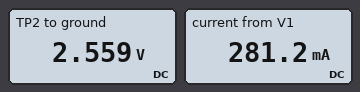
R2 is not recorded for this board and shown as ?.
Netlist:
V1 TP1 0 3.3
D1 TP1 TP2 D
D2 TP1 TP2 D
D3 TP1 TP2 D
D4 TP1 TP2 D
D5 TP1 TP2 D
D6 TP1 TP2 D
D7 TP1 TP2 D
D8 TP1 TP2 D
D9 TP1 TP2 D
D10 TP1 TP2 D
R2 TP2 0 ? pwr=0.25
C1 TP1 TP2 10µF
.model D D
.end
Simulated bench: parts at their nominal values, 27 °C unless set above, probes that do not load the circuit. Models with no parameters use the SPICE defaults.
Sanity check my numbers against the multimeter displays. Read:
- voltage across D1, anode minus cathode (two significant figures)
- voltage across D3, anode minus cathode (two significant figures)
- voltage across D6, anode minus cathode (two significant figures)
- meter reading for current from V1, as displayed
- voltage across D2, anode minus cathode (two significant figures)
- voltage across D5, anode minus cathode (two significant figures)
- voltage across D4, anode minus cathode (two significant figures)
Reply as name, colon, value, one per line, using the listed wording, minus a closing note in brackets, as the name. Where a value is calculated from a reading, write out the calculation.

voltage across D1, anode minus cathode: 3.3 V - 2.559 V = 740 mV
voltage across D3, anode minus cathode: 3.3 V - 2.559 V = 740 mV
voltage across D6, anode minus cathode: 3.3 V - 2.559 V = 740 mV
meter reading for current from V1, as displayed: 281.2 mA
voltage across D2, anode minus cathode: 3.3 V - 2.559 V = 740 mV
voltage across D5, anode minus cathode: 3.3 V - 2.559 V = 740 mV
voltage across D4, anode minus cathode: 3.3 V - 2.559 V = 740 mV
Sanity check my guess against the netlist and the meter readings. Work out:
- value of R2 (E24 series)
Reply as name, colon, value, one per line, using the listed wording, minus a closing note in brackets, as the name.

value of R2: 9.1 Ω
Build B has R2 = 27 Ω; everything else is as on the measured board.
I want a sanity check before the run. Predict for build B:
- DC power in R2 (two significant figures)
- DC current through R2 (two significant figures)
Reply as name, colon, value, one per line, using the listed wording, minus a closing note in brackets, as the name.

DC power in R2: 250 mW
DC current through R2: 96 mA
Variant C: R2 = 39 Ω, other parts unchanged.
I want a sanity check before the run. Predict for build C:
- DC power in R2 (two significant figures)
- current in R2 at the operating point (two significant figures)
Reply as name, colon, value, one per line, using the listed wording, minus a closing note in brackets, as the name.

DC power in R2: 170 mW
current in R2 at the operating point: 67 mA
